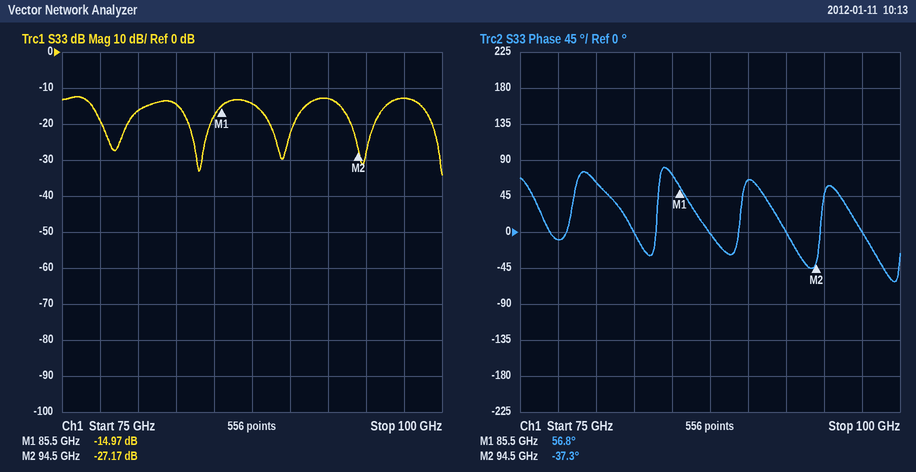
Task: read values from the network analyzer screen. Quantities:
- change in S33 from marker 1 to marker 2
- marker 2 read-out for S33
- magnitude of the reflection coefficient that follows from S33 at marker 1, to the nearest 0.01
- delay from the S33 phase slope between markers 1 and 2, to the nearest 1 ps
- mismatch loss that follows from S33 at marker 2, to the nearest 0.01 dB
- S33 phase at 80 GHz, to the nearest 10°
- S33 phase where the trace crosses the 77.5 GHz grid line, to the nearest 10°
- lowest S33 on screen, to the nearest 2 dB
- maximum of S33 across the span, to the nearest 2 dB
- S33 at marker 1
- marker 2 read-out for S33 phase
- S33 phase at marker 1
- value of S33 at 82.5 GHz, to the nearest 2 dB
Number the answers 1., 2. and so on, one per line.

1. -12.20 dB
2. -27.17 dB
3. 0.18
4. 29 ps
5. 0.01 dB
6. 60°
7. -10°
8. -34 dB
9. -12 dB
10. -14.97 dB
11. -37.3°
12. 56.8°
13. -14 dB
